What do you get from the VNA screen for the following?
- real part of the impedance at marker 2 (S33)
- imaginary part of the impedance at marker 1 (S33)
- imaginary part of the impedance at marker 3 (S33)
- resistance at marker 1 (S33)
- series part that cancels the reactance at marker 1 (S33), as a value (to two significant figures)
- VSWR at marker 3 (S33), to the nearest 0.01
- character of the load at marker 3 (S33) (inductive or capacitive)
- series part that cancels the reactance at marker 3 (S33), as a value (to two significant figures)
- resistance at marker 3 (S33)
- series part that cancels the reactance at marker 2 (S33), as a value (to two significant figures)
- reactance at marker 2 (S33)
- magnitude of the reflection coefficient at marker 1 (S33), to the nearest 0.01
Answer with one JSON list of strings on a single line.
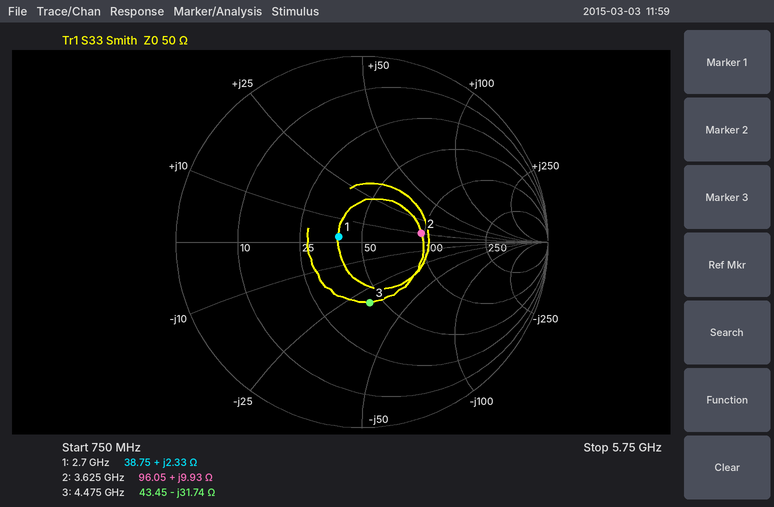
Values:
["96.05 Ω", "+2.33 Ω", "-31.74 Ω", "38.75 Ω", "25 pF", "1.98", "capacitive", "1.1 nH", "43.45 Ω", "4.4 pF", "+9.93 Ω", "0.13"]
